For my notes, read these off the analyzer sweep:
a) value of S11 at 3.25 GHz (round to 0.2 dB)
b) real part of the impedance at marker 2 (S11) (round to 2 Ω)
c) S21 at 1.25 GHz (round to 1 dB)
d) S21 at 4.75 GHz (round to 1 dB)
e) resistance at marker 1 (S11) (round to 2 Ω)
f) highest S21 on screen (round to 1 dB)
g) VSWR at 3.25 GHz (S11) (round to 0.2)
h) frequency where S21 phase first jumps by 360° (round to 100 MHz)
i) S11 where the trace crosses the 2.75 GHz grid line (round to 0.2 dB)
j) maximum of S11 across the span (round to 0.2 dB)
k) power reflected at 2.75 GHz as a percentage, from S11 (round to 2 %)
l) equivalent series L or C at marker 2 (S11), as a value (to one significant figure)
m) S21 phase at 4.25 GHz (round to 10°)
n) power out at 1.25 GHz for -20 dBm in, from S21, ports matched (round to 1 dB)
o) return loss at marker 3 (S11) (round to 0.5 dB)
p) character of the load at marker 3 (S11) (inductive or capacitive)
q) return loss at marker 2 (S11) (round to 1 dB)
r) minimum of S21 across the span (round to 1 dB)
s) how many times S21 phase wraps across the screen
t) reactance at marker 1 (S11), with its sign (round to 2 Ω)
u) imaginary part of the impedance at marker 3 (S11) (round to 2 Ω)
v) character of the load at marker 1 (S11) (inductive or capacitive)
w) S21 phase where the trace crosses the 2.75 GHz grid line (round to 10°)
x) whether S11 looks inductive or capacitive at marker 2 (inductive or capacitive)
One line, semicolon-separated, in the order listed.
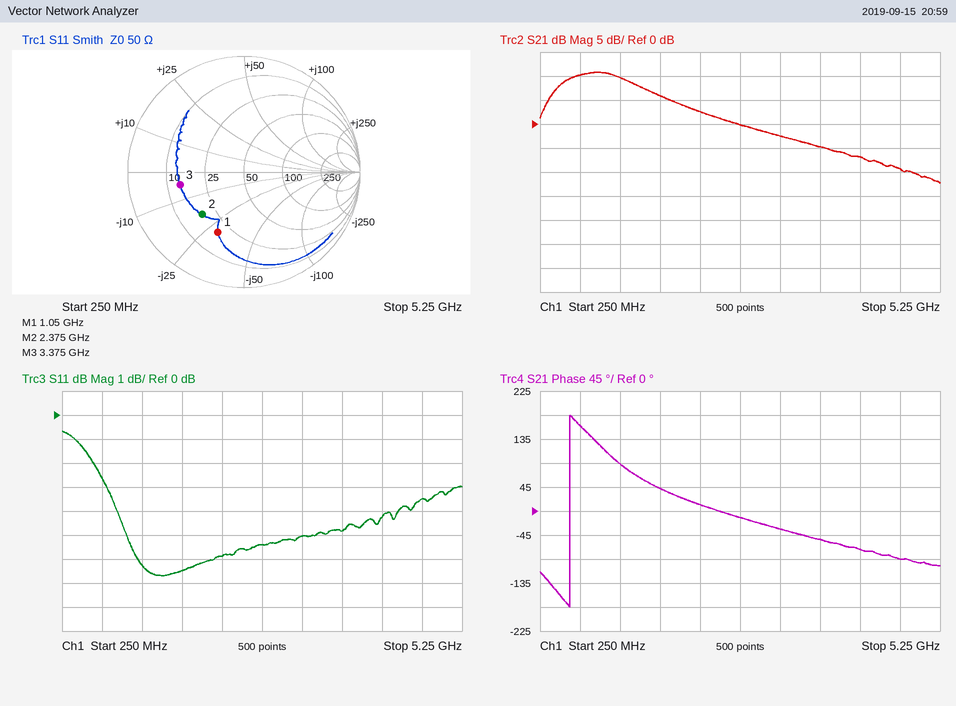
-5.0 dB; 18 Ω; 10 dB; -9 dB; 20 Ω; 11 dB; 3.6; 600 MHz; -5.4 dB; -0.6 dB; 28 %; 4 pF; -70°; -10 dBm; 5.0 dB; capacitive; 6 dB; -12 dB; 1; -30 Ω; -4 Ω; capacitive; -10°; capacitive
